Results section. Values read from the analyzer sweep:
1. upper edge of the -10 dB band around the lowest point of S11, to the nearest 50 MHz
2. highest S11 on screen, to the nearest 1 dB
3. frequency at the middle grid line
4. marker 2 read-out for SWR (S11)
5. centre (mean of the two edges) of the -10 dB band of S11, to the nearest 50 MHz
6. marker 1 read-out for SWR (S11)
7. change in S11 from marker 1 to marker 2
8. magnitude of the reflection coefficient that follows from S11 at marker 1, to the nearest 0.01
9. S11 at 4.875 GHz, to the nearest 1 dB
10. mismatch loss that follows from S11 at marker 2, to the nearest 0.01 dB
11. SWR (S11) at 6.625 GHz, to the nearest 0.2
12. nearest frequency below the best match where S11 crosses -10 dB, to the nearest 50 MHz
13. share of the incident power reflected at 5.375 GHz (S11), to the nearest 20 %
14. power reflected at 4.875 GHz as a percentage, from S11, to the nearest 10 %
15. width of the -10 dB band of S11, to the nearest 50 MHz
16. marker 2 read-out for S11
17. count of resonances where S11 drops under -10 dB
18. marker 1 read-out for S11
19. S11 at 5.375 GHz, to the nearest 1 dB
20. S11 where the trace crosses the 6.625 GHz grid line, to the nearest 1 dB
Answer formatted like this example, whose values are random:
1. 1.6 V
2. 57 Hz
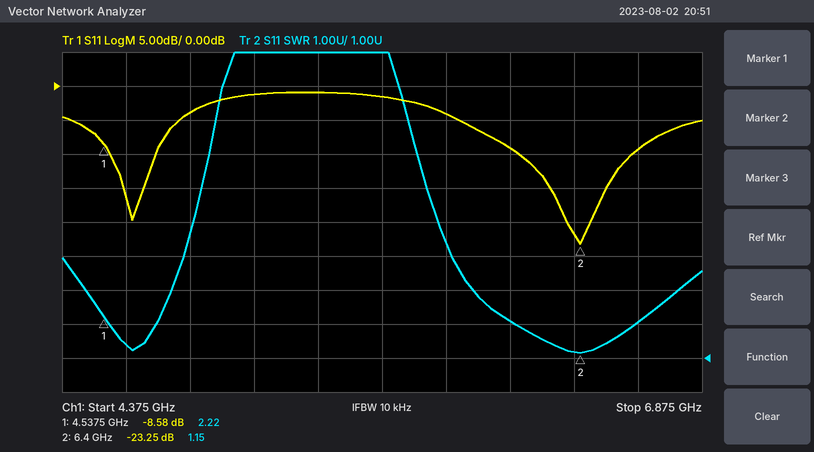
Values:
1. 6.60 GHz
2. -1 dB
3. 5.625 GHz
4. 1.15
5. 6.40 GHz
6. 2.22
7. -14.67 dB
8. 0.37
9. -4 dB
10. 0.02 dB
11. 2.0
12. 6.15 GHz
13. 80 %
14. 40 %
15. 450 MHz
16. -23.25 dB
17. 2
18. -8.58 dB
19. -1 dB
20. -9 dB
